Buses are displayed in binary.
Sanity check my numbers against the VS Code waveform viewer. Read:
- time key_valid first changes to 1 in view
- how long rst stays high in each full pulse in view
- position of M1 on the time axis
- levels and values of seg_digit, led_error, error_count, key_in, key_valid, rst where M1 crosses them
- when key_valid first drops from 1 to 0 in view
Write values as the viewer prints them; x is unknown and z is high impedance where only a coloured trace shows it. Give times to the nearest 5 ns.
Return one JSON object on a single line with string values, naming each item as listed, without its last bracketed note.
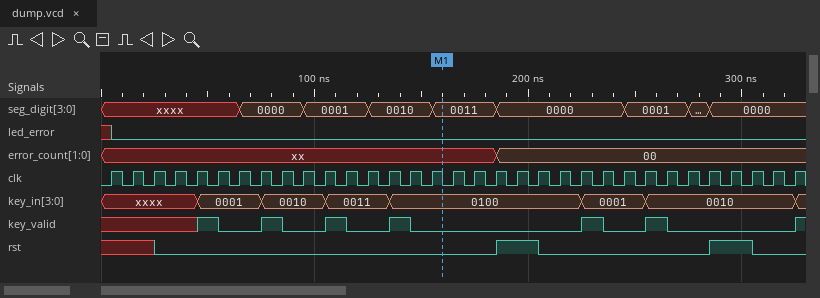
{"time key_valid first changes to 1 in view": "45 ns", "how long rst stays high in each full pulse in view": "20 ns, 20 ns", "position of M1 on the time axis": "160 ns", "levels and values of seg_digit, led_error, error_count, key_in, key_valid, rst where M1 crosses them": "seg_digit=0011, led_error=0, error_count=xx, key_in=0100, key_valid=0, rst=0", "when key_valid first drops from 1 to 0 in view": "55 ns"}
